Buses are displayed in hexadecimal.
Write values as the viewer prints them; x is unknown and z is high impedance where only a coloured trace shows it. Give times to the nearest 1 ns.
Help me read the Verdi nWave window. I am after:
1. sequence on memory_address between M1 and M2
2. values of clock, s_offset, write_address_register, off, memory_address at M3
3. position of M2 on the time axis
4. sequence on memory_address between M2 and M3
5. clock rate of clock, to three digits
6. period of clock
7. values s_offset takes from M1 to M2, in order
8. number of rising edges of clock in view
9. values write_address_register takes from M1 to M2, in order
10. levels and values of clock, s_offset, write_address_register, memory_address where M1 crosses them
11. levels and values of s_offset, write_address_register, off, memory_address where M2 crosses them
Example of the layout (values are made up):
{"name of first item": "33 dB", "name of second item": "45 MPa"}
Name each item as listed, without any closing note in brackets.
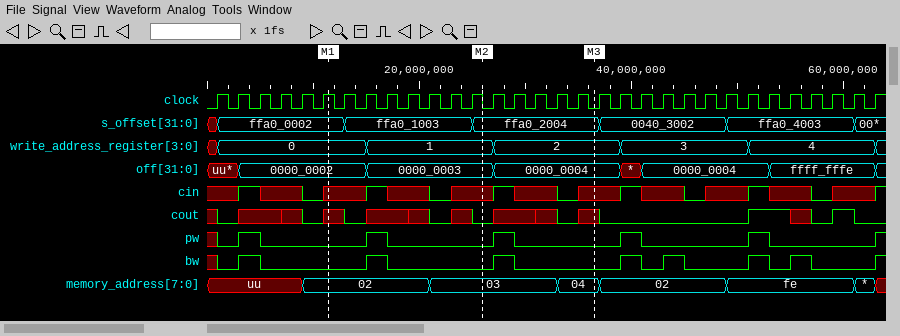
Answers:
{"sequence on memory_address between M1 and M2": "02, 03", "values of clock, s_offset, write_address_register, off, memory_address at M3": "clock=0, s_offset=ffa0_2004, write_address_register=2, off=0000_0004, memory_address=04", "position of M2 on the time axis": "26 ns", "sequence on memory_address between M2 and M3": "03, 04", "clock rate of clock, to three digits": "500 MHz", "period of clock": "2 ns", "values s_offset takes from M1 to M2, in order": "ffa0_0002, ffa0_1003, ffa0_2004", "number of rising edges of clock in view": "32", "values write_address_register takes from M1 to M2, in order": "0, 1", "levels and values of clock, s_offset, write_address_register, memory_address where M1 crosses them": "clock=1, s_offset=ffa0_0002, write_address_register=0, memory_address=02", "levels and values of s_offset, write_address_register, off, memory_address where M2 crosses them": "s_offset=ffa0_2004, write_address_register=1, off=0000_0003, memory_address=03"}
